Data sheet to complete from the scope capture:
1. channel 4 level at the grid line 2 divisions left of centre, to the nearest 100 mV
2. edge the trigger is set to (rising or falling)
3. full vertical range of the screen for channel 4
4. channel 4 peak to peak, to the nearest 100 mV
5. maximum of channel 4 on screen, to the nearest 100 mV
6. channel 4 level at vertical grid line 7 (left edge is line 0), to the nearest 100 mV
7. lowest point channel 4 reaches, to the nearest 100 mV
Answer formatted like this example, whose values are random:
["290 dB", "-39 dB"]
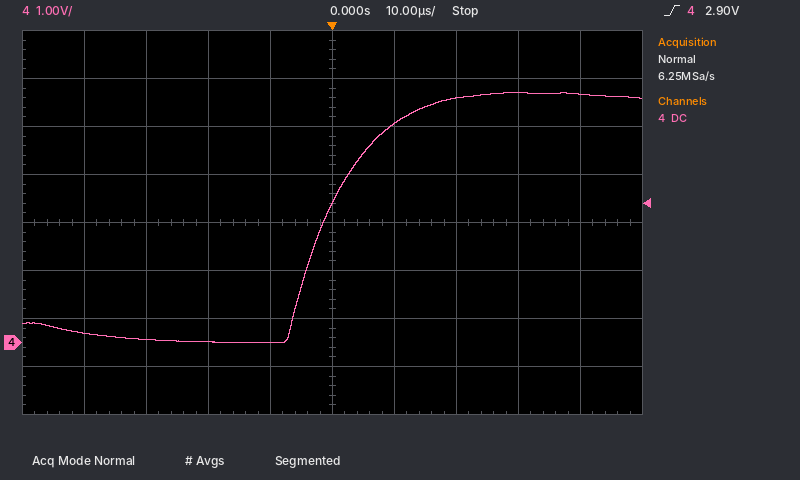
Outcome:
["0.0 V", "rising", "8 V", "5.2 V", "5.2 V", "5.1 V", "0.0 V"]
